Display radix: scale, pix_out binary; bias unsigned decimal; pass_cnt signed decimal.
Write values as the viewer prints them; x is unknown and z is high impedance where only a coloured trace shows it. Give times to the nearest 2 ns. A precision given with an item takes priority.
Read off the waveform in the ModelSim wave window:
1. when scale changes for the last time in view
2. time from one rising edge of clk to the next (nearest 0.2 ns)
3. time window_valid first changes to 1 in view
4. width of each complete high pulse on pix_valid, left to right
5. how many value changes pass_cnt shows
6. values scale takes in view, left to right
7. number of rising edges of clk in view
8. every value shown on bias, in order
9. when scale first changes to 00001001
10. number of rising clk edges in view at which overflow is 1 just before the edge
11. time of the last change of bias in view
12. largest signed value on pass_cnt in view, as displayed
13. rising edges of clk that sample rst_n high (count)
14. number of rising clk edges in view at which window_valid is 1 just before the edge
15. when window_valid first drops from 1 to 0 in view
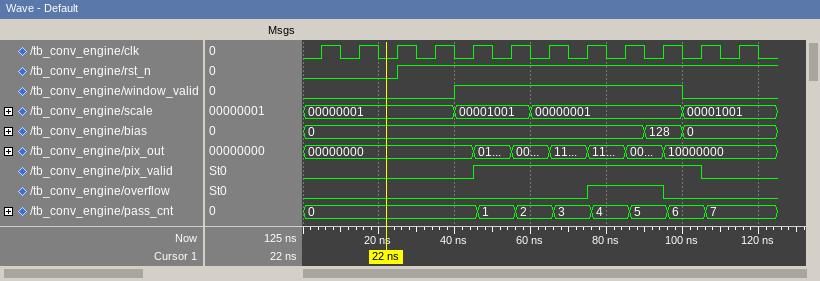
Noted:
100 ns
10 ns
40 ns
60 ns
7
00000001, 00001001, 00000001, 00001001
12
0, 128, 0
40 ns
2
100 ns
7
9
6
100 ns
